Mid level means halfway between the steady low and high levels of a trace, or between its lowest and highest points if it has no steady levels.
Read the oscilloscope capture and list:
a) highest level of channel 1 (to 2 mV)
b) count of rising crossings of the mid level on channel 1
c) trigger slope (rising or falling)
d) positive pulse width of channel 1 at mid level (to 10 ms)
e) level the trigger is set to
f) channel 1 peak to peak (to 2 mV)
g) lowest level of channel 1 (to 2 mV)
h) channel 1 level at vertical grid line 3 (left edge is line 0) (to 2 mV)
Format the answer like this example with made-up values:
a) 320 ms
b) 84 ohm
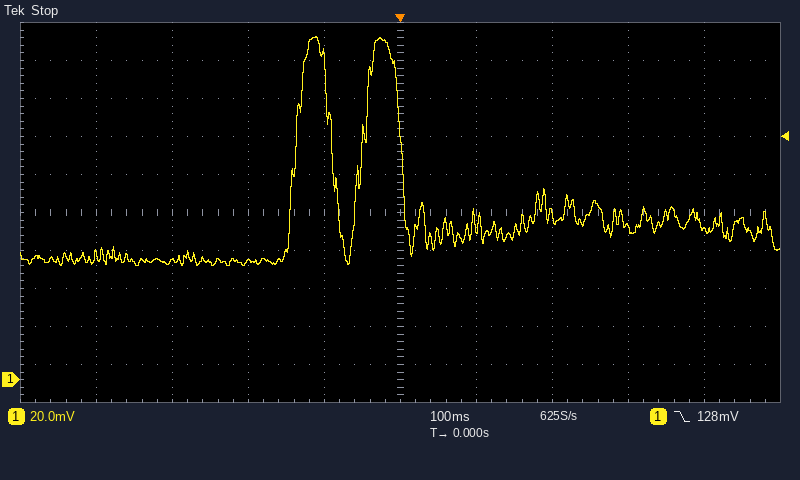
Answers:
a) 180 mV
b) 2
c) falling
d) 50 ms
e) 128 mV
f) 120 mV
g) 60 mV
h) 62 mV
